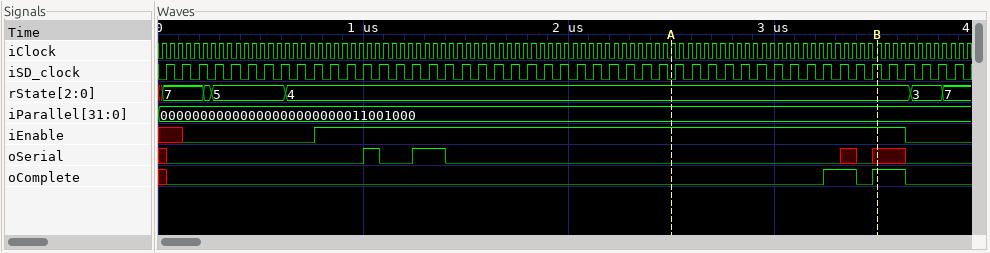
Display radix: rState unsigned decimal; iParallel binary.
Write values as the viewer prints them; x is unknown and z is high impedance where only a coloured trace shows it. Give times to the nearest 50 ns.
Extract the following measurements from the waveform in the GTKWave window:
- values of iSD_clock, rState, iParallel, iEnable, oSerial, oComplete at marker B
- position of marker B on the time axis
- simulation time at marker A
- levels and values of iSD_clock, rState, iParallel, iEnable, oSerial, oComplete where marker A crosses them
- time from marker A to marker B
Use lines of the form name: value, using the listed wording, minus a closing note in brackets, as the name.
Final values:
values of iSD_clock, rState, iParallel, iEnable, oSerial, oComplete at marker B: iSD_clock=1, rState=4, iParallel=00000000000000000000000011001000, iEnable=1, oSerial=x, oComplete=1
position of marker B on the time axis: 3500 ns
simulation time at marker A: 2500 ns
levels and values of iSD_clock, rState, iParallel, iEnable, oSerial, oComplete where marker A crosses them: iSD_clock=0, rState=4, iParallel=00000000000000000000000011001000, iEnable=1, oSerial=0, oComplete=0
time from marker A to marker B: 1000 ns
